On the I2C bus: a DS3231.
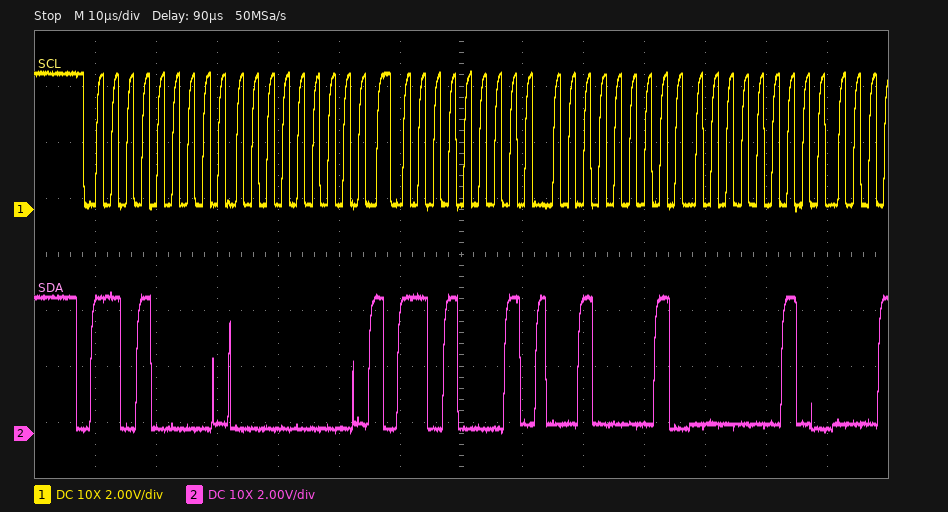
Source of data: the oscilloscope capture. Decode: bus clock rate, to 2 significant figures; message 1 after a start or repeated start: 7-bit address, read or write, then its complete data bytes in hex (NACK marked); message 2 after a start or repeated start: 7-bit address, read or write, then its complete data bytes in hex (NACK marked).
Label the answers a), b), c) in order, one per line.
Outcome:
a) 400 kHz
b) 0x68 write: 00
c) 0x68 read: 21 02
